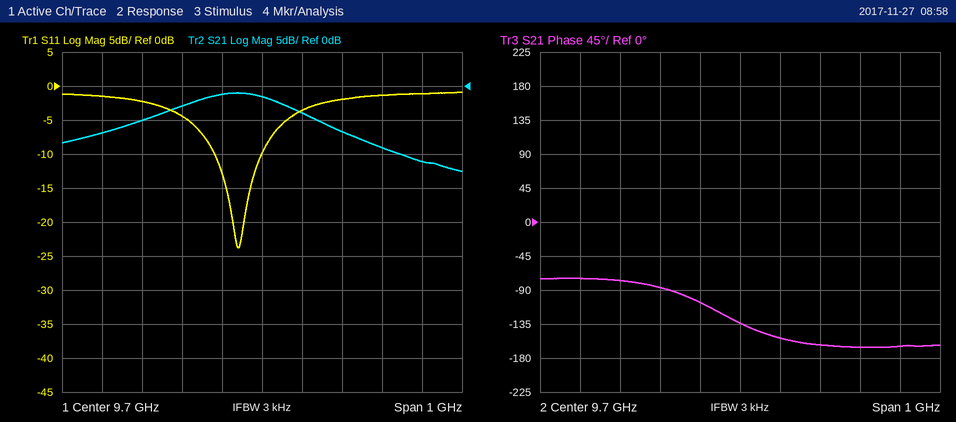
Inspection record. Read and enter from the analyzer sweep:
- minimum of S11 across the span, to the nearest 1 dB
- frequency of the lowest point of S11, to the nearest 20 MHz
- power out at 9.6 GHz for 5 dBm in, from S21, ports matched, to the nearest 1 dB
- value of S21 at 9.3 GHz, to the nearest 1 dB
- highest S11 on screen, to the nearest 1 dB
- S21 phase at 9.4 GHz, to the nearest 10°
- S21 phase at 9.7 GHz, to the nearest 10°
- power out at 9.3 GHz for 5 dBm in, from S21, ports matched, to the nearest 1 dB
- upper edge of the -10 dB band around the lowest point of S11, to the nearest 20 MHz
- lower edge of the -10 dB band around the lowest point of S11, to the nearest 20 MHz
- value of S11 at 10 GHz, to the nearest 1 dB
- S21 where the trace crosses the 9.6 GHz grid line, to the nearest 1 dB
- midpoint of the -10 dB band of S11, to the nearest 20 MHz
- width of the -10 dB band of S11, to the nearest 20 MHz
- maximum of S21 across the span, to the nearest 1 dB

-24 dB
9.64 GHz
4 dBm
-7 dB
-1 dB
-80°
-130°
-2 dBm
9.70 GHz
9.58 GHz
-1 dB
-1 dB
9.64 GHz
120 MHz
-1 dB
